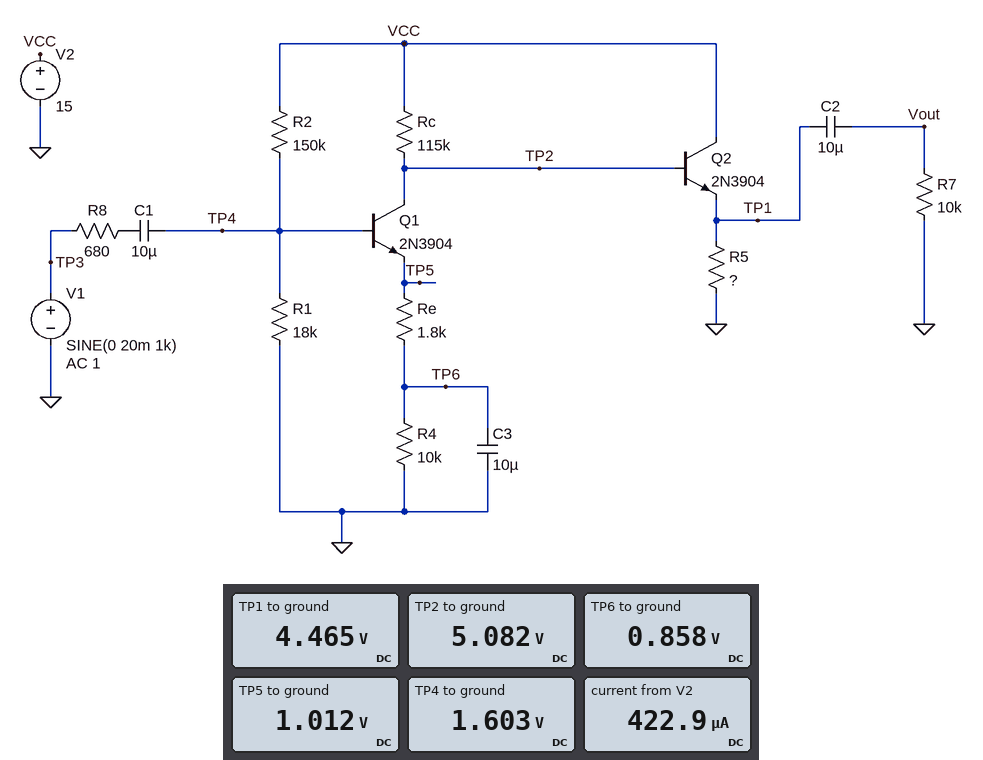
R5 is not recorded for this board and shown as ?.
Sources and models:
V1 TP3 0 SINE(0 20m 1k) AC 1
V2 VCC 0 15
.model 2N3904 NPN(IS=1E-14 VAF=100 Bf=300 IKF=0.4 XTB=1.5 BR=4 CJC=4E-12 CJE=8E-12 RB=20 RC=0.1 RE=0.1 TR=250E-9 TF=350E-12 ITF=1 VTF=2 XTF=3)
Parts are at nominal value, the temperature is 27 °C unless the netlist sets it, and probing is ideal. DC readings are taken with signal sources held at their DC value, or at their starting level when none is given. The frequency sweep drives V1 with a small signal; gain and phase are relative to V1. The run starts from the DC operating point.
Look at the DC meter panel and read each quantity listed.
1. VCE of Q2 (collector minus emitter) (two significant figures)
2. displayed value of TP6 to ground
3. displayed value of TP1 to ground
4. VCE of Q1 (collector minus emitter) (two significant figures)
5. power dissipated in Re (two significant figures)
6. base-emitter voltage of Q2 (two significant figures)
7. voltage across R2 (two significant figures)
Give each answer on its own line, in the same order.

11 V
0.858 V
4.465 V
4.1 V
13 µW
620 mV
13 V
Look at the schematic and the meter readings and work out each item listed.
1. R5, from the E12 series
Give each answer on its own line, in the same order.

18 kΩ
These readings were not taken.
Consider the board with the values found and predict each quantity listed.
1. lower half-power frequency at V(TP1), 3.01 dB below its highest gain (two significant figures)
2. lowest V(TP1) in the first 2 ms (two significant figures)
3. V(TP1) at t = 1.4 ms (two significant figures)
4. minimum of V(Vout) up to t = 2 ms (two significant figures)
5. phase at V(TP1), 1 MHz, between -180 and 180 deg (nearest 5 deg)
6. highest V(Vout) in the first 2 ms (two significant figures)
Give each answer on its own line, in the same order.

8.9 Hz
3.5 V
3.9 V
-950 mV
105 deg
970 mV
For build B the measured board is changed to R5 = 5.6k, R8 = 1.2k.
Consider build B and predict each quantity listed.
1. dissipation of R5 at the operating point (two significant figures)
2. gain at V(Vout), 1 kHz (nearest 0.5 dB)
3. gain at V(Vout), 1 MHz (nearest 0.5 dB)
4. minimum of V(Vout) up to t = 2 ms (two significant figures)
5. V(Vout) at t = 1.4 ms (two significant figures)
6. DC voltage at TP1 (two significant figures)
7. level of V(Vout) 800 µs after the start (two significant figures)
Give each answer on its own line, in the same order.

3.2 mW
33.0 dB
22.0 dB
-900 mV
-520 mV
4.3 V
860 mV
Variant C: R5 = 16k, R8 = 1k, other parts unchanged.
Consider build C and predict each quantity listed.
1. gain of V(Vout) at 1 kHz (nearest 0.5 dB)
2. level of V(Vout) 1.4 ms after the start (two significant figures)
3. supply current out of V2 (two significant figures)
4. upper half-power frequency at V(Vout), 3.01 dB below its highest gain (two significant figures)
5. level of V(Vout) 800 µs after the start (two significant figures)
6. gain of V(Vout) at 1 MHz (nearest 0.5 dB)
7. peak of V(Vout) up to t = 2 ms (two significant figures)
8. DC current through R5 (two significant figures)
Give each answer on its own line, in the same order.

33.5 dB
-540 mV
450 µA
280 kHz
900 mV
22.0 dB
950 mV
280 µA
